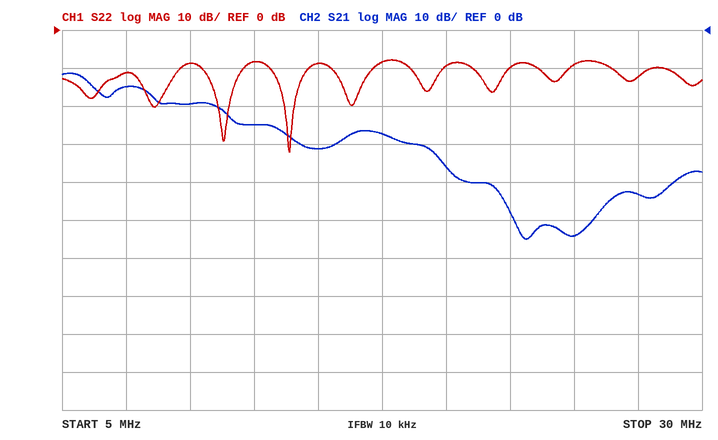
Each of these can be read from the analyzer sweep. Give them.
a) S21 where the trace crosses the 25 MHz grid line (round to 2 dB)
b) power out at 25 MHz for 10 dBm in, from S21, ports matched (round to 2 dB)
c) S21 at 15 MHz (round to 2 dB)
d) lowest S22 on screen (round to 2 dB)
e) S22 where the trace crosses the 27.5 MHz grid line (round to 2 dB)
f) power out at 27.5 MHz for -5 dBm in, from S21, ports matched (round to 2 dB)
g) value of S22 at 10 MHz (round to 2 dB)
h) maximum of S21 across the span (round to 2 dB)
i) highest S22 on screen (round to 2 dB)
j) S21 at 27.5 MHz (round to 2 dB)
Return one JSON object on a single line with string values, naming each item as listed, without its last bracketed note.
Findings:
{"S21 where the trace crosses the 25 MHz grid line": "-54 dB", "power out at 25 MHz for 10 dBm in, from S21, ports matched": "-44 dBm", "S21 at 15 MHz": "-32 dB", "lowest S22 on screen": "-32 dB", "S22 where the trace crosses the 27.5 MHz grid line": "-12 dB", "power out at 27.5 MHz for -5 dBm in, from S21, ports matched": "-48 dBm", "value of S22 at 10 MHz": "-8 dB", "maximum of S21 across the span": "-12 dB", "highest S22 on screen": "-8 dB", "S21 at 27.5 MHz": "-44 dB"}
